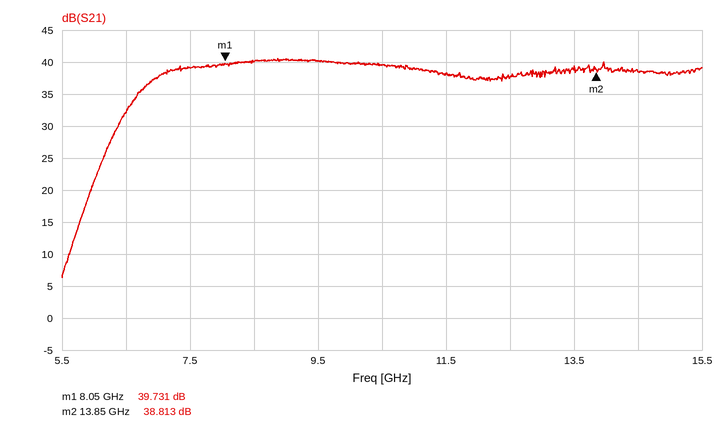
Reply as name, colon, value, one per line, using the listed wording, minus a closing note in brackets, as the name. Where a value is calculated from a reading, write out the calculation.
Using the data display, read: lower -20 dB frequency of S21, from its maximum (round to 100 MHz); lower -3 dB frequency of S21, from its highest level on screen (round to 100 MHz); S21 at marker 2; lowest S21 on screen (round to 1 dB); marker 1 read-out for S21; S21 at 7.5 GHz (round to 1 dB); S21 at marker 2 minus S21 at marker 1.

lower -20 dB frequency of S21, from its maximum: 6.0 GHz
lower -3 dB frequency of S21, from its highest level on screen: 7.0 GHz
S21 at marker 2: 38.813 dB
lowest S21 on screen: 6 dB
marker 1 read-out for S21: 39.731 dB
S21 at 7.5 GHz: 39 dB
S21 at marker 2 minus S21 at marker 1: 38.813 − (39.731) = -0.918 dB
